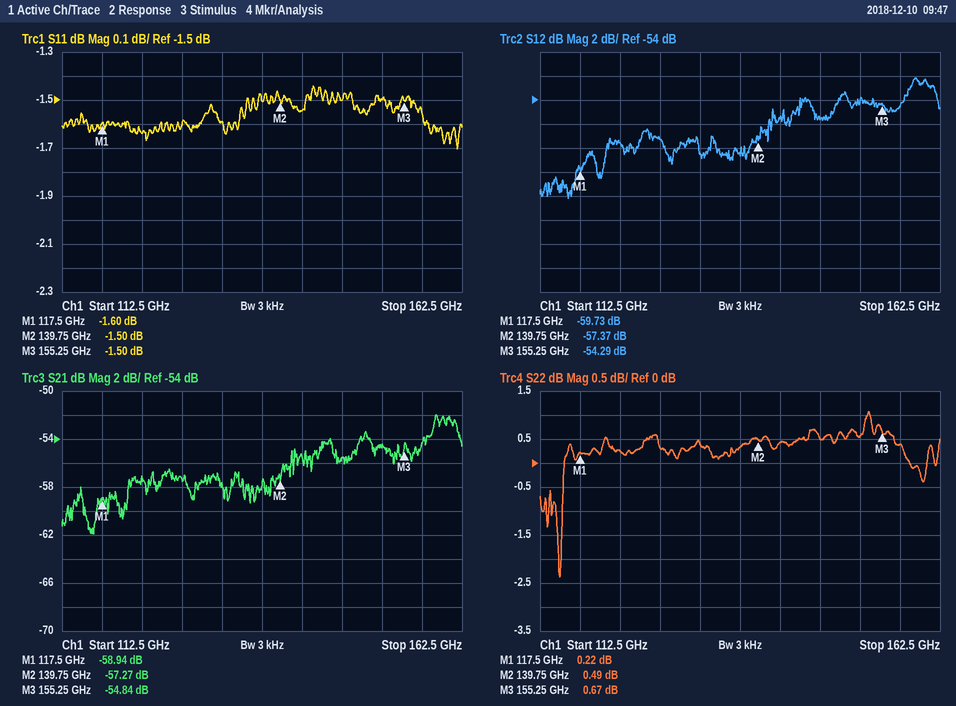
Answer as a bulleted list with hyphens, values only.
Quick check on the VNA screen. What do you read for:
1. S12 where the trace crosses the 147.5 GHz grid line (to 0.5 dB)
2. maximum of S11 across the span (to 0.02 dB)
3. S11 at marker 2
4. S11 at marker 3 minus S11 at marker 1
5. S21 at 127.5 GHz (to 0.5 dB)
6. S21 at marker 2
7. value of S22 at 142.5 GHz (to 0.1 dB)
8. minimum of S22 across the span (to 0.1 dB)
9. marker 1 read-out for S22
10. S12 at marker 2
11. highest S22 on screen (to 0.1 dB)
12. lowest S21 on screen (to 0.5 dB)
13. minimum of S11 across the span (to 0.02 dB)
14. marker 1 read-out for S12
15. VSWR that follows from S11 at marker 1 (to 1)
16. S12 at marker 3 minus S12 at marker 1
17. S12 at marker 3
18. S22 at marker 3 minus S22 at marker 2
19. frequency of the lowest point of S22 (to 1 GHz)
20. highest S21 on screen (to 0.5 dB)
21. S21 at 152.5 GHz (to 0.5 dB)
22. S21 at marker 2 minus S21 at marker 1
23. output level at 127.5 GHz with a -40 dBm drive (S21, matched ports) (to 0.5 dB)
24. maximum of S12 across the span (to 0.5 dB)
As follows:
- -55.5 dB
- -1.44 dB
- -1.50 dB
- 0.10 dB
- -57.5 dB
- -57.27 dB
- 0.4 dB
- -2.4 dB
- 0.22 dB
- -57.37 dB
- 1.1 dB
- -62.0 dB
- -1.70 dB
- -59.73 dB
- 11
- 5.44 dB
- -54.29 dB
- 0.18 dB
- 115 GHz
- -52.0 dB
- -54.5 dB
- 1.67 dB
- -97.5 dBm
- -52.0 dB
